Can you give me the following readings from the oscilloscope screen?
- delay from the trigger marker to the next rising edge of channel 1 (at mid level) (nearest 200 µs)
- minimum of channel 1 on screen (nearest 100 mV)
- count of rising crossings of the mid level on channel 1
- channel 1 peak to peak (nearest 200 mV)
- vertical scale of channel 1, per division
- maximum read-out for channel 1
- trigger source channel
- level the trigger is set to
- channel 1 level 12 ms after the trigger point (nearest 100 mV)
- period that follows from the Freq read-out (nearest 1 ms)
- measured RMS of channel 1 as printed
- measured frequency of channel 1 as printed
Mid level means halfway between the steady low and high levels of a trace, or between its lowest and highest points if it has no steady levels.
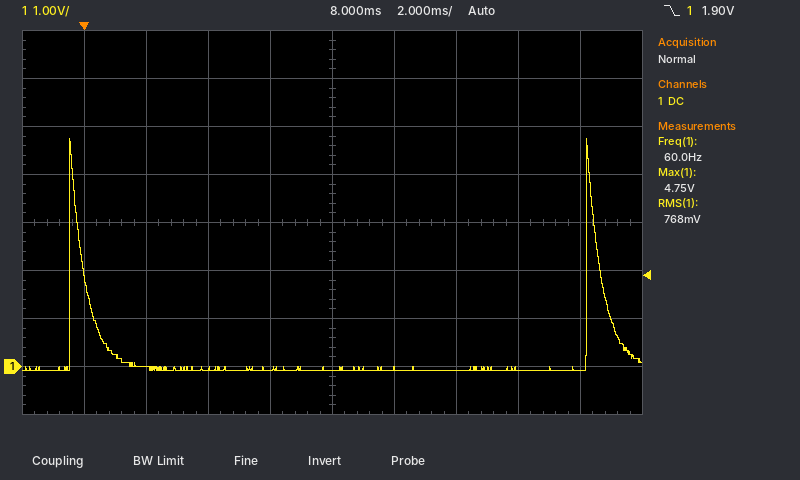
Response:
16.2 ms
-100 mV
2
4.8 V
1 V
4.75 V
channel 1
1.90 V
-100 mV
17 ms
768 mV
60.0 Hz
